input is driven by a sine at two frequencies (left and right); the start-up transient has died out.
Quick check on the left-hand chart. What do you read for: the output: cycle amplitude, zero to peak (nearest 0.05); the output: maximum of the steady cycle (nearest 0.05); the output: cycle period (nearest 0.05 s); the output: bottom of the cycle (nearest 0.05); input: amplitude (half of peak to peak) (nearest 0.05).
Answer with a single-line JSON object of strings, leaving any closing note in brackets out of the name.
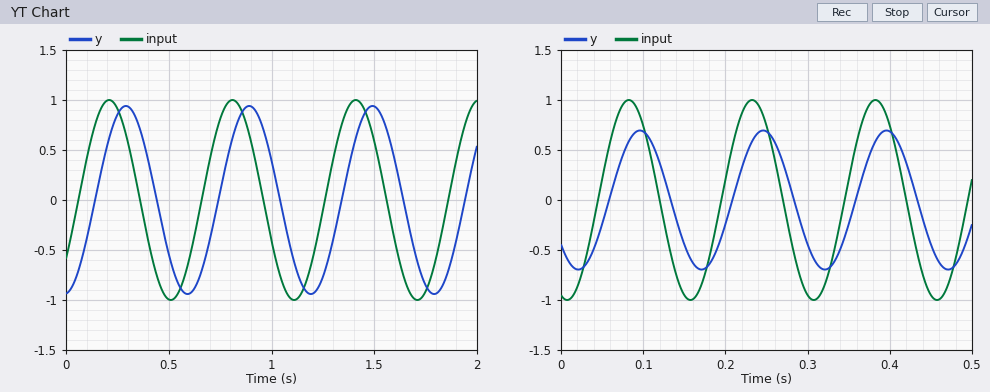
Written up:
{"the output: cycle amplitude, zero to peak": "0.95", "the output: maximum of the steady cycle": "0.95", "the output: cycle period": "0.60 s", "the output: bottom of the cycle": "-0.95", "input: amplitude (half of peak to peak)": "1.00"}
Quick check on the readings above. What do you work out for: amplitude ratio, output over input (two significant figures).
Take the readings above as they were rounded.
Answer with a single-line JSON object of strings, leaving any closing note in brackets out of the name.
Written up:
{"amplitude ratio, output over input": "0.95"}
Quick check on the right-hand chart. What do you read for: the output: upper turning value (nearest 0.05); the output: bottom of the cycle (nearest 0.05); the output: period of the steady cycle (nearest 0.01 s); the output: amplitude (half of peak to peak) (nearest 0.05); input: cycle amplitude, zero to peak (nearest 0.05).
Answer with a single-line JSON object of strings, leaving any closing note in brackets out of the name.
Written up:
{"the output: upper turning value": "0.70", "the output: bottom of the cycle": "-0.70", "the output: period of the steady cycle": "0.15 s", "the output: amplitude (half of peak to peak)": "0.70", "input: cycle amplitude, zero to peak": "1.00"}
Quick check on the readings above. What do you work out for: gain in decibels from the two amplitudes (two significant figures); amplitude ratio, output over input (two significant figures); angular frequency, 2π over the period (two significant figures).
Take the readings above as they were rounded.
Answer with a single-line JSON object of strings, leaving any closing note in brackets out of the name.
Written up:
{"gain in decibels from the two amplitudes": "-3.1 dB", "amplitude ratio, output over input": "0.70", "angular frequency, 2π over the period": "42 rad/s"}
